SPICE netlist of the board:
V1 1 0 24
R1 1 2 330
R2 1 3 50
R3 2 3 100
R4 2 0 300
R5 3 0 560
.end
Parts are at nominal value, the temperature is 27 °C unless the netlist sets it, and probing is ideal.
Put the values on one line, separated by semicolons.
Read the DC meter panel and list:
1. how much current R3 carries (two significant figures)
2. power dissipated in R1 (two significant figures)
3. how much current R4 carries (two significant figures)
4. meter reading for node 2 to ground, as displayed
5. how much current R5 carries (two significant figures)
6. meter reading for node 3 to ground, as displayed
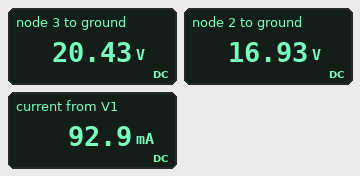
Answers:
35 mA; 150 mW; 56 mA; 16.93 V; 36 mA; 20.43 V
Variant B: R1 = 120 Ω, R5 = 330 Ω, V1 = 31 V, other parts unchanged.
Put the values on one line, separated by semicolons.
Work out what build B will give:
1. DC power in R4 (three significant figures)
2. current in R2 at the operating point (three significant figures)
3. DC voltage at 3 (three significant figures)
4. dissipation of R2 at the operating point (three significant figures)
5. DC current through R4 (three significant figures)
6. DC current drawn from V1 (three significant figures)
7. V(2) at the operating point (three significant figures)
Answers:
1.91 W; 99.7 mA; 26.0 V; 497 mW; 79.8 mA; 159 mA; 23.9 V
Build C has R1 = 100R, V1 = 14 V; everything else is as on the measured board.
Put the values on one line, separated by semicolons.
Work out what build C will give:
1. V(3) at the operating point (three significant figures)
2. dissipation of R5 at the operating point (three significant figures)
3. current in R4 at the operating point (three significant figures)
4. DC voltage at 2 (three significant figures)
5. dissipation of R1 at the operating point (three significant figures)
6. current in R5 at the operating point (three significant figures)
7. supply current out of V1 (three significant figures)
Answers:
12.4 V; 273 mW; 37.7 mA; 11.3 V; 73.0 mW; 22.1 mA; 59.7 mA
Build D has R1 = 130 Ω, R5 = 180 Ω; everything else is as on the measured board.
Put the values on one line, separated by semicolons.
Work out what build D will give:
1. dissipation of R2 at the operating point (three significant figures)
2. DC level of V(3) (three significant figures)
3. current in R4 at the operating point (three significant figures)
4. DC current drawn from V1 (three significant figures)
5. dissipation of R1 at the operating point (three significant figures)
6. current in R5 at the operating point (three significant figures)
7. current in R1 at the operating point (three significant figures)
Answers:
619 mW; 18.4 V; 58.5 mA; 161 mA; 320 mW; 102 mA; 49.6 mA
